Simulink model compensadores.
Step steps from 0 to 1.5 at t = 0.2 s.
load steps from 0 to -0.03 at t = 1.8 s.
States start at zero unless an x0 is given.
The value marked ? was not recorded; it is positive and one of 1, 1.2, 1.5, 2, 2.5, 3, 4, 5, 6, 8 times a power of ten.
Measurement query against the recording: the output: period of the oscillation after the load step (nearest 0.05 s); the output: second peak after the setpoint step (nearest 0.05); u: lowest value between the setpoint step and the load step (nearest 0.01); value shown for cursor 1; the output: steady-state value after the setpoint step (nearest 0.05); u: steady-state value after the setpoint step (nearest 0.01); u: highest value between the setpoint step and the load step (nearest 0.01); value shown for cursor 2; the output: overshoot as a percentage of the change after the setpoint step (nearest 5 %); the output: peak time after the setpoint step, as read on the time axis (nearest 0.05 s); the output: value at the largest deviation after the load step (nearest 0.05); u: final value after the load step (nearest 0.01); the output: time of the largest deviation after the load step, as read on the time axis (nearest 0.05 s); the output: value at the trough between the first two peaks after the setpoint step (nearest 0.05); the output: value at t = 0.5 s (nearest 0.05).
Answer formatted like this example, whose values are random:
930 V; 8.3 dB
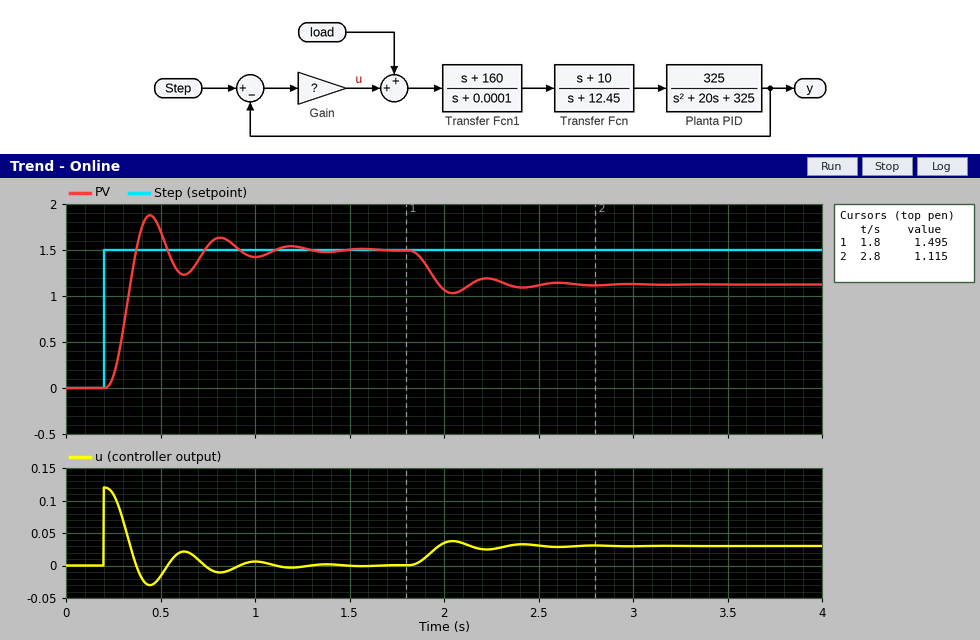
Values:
0.35 s; 1.65; -0.03; 1.495; 1.50; 0.00; 0.12; 1.115; 25 %; 0.45 s; 1.05; 0.03; 2.05 s; 1.25; 1.70
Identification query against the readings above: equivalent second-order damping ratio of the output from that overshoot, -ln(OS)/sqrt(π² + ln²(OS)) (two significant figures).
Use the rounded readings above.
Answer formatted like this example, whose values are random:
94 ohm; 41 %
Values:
0.40
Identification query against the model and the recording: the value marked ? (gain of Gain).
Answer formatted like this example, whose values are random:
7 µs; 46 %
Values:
0.08
